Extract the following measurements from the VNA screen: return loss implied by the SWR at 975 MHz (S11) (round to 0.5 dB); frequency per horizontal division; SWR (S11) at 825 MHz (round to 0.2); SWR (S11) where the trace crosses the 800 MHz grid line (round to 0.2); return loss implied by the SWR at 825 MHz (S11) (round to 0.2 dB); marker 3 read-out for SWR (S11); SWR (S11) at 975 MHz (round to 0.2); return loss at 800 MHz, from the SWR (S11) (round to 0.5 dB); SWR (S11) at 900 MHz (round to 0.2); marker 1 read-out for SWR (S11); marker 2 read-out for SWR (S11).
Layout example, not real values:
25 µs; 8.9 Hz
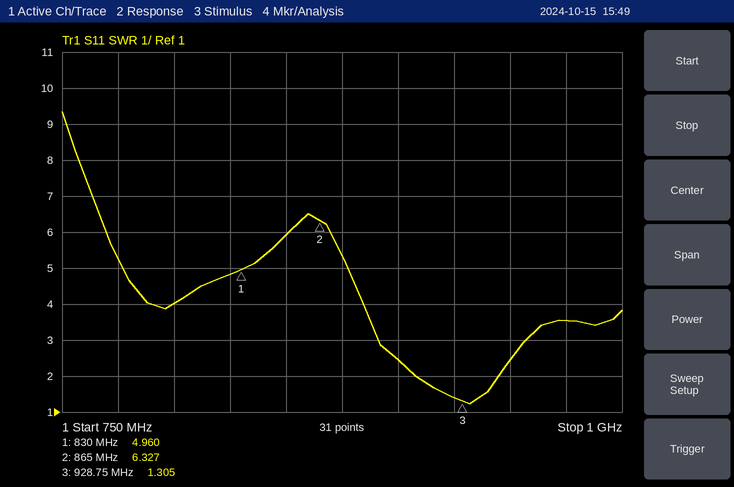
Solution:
5.0 dB; 25 MHz; 4.8; 4.0; 3.6 dB; 1.305; 3.6; 4.5 dB; 2.4; 4.960; 6.327
